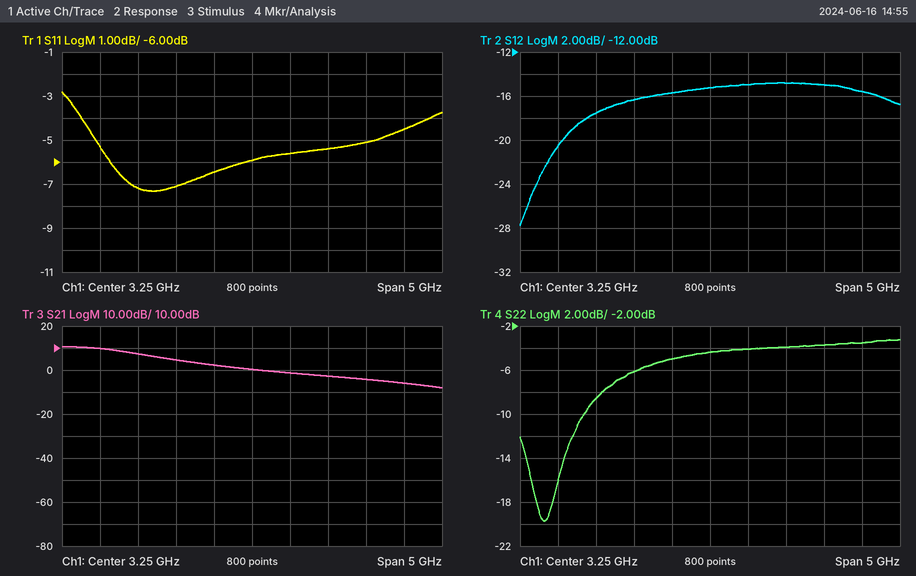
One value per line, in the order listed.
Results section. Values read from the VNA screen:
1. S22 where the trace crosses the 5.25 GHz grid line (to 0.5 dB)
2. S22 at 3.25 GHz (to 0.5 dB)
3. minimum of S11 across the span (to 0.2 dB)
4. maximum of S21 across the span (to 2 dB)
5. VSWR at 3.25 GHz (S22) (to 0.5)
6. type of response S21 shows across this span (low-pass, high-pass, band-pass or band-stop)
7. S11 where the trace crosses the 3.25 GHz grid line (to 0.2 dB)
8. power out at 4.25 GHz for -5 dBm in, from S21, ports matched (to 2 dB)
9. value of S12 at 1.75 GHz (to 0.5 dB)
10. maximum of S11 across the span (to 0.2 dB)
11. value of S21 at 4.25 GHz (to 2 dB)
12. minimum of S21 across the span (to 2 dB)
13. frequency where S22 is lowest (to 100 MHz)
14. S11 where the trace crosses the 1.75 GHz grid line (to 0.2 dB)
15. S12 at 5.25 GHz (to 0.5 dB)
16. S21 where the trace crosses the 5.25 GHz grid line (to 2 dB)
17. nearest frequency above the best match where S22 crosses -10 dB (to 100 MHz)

-3.5 dB
-4.5 dB
-7.4 dB
10 dB
4.0
low-pass
-6.0 dB
-8 dBm
-17.5 dB
-2.8 dB
-2 dB
-8 dB
1.1 GHz
-7.2 dB
-15.5 dB
-6 dB
1.6 GHz
